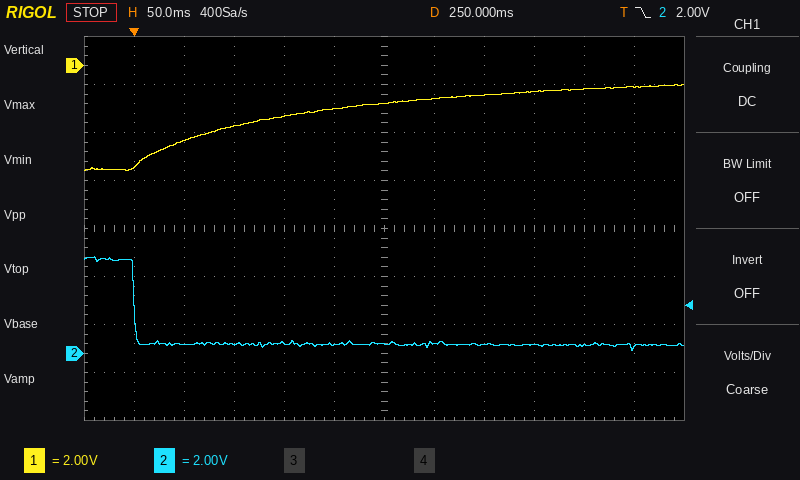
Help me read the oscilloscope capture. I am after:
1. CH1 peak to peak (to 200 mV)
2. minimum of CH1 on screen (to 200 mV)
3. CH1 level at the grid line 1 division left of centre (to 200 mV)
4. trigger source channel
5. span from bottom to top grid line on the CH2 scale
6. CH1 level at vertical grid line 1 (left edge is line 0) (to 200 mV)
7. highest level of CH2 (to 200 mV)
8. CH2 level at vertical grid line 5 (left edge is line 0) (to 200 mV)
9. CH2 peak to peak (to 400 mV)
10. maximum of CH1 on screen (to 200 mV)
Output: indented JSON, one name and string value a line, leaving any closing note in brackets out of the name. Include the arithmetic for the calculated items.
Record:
{
  "CH1 peak to peak": "-800 mV − (-4.4 V) = 3.6 V",
  "minimum of CH1 on screen": "-4.4 V",
  "CH1 level at the grid line 1 division left of centre": "-1.8 V",
  "trigger source channel": "CH2",
  "span from bottom to top grid line on the CH2 scale": "16 V",
  "CH1 level at vertical grid line 1 (left edge is line 0)": "-4.2 V",
  "highest level of CH2": "4.0 V",
  "CH2 level at vertical grid line 5 (left edge is line 0)": "400 mV",
  "CH2 peak to peak": "4.0 V",
  "maximum of CH1 on screen": "-800 mV"
}
